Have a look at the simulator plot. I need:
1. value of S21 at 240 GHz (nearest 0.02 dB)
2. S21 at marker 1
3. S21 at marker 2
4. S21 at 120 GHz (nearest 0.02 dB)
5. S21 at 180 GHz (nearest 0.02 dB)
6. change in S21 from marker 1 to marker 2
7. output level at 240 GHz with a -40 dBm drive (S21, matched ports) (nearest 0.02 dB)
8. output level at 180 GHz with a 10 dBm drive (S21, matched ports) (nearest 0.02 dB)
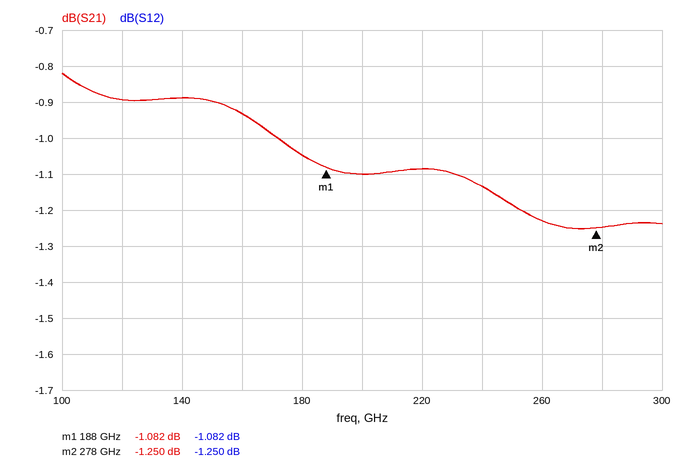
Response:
-1.14 dB
-1.082 dB
-1.250 dB
-0.90 dB
-1.04 dB
-0.168 dB
-41.14 dBm
8.96 dBm
